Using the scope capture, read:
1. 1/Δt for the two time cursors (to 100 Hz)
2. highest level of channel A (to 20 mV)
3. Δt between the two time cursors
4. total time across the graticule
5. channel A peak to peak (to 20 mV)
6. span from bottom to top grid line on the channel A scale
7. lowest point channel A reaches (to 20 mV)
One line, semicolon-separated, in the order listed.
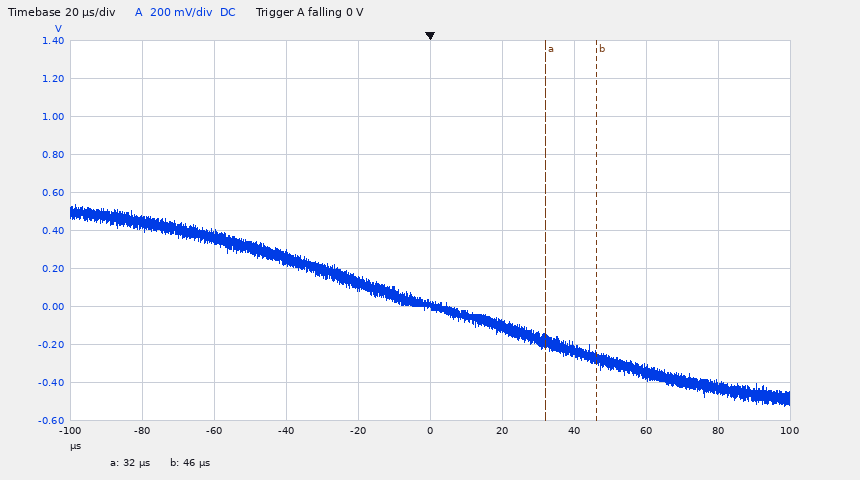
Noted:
71.4 kHz; 540 mV; 14 µs; 200 µs; 1.06 V; 2 V; -520 mV
